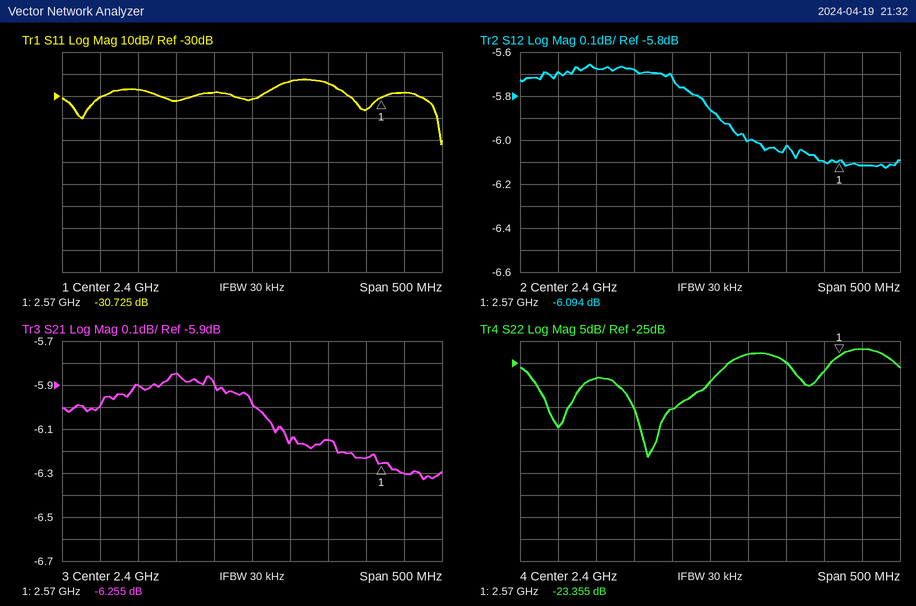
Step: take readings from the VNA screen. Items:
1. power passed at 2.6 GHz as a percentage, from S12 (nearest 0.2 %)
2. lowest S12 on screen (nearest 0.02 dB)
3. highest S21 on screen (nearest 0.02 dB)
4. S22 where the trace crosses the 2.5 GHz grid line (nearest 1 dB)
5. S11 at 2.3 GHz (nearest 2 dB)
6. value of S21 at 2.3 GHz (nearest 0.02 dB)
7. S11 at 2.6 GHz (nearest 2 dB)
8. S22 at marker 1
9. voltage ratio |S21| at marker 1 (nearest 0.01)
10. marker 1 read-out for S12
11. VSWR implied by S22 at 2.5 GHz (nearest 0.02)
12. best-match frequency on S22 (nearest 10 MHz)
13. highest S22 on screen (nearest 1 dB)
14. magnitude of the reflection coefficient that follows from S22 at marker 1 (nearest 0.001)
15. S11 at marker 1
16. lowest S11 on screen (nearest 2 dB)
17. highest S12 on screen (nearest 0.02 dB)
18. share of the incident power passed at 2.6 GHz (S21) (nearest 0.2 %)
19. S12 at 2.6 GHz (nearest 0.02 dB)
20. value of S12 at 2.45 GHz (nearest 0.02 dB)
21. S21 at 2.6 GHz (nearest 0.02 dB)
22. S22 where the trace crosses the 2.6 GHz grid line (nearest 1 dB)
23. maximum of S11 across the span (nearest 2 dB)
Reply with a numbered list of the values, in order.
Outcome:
1. 24.4 %
2. -6.12 dB
3. -5.84 dB
4. -25 dB
5. -32 dB
6. -5.84 dB
7. -28 dB
8. -23.355 dB
9. 0.49
10. -6.094 dB
11. 1.12
12. 2.32 GHz
13. -22 dB
14. 0.068
15. -30.725 dB
16. -52 dB
17. -5.66 dB
18. 23.4 %
19. -6.12 dB
20. -6.00 dB
21. -6.30 dB
22. -22 dB
23. -22 dB
